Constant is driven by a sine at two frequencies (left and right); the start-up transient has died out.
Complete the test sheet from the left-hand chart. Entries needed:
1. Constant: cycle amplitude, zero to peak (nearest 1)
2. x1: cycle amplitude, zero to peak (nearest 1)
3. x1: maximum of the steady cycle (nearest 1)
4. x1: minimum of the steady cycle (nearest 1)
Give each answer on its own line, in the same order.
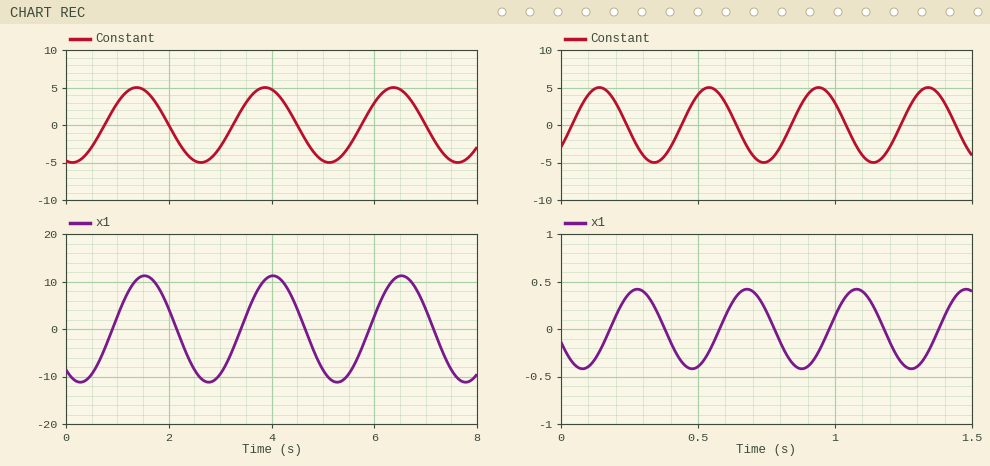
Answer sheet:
5
11
11
-11
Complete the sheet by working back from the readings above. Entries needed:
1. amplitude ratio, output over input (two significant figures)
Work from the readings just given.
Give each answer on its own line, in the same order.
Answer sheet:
2.2
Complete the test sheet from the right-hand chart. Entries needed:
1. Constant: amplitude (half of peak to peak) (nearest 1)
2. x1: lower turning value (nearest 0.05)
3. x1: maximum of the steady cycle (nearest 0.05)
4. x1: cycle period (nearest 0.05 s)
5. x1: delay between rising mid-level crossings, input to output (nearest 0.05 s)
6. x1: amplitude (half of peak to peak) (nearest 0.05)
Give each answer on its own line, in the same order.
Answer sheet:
5
-0.40
0.40
0.40 s
0.15 s
0.40
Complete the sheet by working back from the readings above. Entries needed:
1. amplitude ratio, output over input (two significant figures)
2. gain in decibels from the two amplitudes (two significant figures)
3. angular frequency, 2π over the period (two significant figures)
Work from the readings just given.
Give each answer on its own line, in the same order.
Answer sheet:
0.080
-22 dB
16 rad/s
